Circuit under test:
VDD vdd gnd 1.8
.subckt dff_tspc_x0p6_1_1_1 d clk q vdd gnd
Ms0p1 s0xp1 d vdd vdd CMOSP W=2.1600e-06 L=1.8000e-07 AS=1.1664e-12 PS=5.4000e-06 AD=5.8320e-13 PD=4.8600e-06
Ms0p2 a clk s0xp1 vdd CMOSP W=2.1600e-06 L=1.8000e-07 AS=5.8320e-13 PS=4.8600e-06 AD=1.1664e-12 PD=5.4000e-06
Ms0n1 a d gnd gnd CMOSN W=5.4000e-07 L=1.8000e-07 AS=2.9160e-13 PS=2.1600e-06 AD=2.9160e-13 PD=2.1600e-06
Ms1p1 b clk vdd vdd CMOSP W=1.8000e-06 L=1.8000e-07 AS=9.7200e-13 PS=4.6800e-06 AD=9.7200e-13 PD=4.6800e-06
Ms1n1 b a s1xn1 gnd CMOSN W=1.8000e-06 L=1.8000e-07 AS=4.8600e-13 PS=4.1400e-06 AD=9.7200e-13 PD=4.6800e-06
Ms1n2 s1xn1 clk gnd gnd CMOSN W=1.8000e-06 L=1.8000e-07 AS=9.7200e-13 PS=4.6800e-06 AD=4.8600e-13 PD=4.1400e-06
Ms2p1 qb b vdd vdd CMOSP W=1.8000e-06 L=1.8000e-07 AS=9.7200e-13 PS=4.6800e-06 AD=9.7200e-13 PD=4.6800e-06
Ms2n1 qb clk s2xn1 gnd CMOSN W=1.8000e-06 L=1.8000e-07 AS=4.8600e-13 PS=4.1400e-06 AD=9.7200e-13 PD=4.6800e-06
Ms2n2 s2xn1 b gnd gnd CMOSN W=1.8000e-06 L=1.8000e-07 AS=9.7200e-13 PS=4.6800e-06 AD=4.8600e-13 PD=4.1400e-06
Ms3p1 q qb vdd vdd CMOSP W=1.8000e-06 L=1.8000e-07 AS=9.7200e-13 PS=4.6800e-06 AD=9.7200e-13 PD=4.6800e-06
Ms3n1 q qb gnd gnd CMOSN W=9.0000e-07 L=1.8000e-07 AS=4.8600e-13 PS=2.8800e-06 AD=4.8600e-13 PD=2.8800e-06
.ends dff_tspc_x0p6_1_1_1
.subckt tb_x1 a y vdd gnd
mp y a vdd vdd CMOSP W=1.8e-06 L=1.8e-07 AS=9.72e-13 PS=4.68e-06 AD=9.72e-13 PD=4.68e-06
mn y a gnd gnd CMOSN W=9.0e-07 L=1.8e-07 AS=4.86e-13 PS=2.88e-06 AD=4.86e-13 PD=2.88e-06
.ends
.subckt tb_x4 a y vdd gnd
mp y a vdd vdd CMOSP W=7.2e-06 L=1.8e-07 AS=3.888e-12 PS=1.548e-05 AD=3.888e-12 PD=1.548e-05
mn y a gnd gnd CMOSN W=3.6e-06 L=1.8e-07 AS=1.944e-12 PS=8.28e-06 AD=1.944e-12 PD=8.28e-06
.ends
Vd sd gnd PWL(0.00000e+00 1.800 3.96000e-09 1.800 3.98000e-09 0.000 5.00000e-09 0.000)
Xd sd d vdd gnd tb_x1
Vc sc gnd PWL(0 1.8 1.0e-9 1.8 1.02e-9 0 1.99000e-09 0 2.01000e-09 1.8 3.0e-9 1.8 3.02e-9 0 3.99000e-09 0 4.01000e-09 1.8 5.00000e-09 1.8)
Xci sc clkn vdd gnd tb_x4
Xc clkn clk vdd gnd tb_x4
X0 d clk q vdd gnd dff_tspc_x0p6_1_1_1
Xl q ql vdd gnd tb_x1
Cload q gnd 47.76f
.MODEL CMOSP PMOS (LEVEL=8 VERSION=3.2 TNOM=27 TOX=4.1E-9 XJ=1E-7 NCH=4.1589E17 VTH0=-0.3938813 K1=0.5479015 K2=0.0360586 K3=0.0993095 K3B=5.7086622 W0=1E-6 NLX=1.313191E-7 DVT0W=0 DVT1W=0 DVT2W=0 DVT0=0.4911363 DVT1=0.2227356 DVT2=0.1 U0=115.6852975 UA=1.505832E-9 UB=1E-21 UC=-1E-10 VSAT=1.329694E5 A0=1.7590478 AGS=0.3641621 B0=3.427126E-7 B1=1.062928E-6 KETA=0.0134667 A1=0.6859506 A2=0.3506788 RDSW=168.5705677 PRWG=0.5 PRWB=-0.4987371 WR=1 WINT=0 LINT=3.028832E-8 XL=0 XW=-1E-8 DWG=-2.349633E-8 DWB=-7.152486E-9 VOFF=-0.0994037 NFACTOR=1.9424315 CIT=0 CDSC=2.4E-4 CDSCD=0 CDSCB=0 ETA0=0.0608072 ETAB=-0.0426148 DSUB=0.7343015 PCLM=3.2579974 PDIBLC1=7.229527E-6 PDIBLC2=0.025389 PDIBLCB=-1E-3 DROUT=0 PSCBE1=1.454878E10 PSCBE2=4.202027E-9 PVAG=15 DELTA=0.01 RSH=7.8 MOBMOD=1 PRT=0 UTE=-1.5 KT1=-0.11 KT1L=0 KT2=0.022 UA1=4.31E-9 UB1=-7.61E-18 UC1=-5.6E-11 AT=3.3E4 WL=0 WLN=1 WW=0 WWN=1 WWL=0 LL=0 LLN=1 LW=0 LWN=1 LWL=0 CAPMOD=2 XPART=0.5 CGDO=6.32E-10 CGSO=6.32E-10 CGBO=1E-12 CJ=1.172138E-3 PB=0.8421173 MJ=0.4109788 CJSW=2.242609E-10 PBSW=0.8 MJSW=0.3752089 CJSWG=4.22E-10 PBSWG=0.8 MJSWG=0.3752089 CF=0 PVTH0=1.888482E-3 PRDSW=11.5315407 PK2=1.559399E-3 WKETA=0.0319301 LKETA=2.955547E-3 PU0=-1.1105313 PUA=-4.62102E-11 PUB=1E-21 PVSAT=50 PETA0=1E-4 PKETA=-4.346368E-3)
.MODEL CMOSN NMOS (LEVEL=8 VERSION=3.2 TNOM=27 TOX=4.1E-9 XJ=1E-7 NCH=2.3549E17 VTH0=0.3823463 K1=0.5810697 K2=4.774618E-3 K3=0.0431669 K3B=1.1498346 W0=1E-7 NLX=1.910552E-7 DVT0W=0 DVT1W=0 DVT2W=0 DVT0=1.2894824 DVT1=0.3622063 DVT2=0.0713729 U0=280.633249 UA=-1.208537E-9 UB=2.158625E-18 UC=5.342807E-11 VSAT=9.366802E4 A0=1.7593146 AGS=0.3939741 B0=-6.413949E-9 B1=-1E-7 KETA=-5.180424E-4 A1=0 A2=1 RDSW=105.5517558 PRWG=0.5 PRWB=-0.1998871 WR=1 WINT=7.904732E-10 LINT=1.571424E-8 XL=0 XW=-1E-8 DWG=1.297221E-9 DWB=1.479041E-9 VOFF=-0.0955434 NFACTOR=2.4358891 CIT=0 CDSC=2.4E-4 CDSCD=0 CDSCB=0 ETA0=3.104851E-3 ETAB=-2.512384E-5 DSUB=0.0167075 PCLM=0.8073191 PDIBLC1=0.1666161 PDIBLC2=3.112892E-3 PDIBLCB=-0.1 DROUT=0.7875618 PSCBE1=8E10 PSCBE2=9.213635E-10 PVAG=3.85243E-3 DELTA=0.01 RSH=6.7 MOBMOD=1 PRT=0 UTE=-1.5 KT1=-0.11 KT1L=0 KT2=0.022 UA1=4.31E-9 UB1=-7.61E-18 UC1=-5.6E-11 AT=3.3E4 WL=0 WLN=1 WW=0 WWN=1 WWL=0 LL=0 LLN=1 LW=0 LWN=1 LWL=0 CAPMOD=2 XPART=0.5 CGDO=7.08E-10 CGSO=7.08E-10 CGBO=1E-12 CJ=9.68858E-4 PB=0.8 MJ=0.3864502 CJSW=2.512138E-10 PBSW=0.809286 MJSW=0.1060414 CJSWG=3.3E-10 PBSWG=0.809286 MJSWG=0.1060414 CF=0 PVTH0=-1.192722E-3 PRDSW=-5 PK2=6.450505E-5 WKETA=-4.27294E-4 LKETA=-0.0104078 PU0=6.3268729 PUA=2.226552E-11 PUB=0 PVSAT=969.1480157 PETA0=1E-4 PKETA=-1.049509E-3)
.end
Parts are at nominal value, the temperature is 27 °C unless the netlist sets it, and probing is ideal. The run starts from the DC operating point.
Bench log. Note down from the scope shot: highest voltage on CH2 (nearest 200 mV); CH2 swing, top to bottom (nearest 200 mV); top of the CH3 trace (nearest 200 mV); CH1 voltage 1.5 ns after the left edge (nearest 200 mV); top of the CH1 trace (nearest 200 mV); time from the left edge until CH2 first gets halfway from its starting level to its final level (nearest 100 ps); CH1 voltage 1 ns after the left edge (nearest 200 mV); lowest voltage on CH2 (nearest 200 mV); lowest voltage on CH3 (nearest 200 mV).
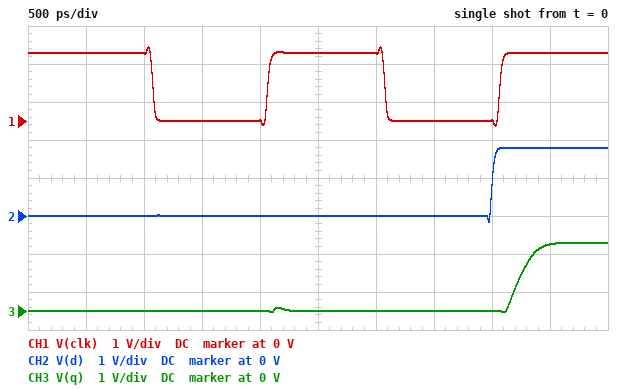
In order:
1.8 V
2.0 V
1.8 V
0 V
2.0 V
4.0 ns
1.8 V
-200 mV
0 V
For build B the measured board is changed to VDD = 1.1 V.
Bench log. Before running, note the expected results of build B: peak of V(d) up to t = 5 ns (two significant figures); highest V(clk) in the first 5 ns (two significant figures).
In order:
1.1 V
1.2 V
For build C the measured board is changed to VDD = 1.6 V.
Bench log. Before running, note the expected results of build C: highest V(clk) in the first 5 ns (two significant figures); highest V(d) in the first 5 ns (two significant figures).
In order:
1.7 V
1.6 V
